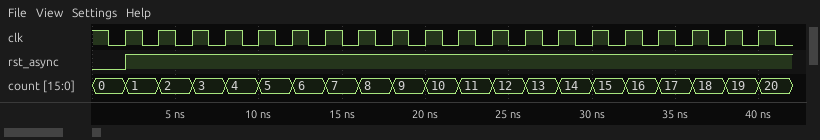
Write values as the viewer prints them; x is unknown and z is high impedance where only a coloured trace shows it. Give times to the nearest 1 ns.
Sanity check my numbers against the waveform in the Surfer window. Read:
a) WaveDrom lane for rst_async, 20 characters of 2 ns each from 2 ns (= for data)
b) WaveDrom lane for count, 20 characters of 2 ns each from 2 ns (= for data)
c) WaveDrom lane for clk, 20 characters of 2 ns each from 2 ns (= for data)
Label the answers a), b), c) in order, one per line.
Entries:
a) {name: 'rst_async', wave: '1...................'}
b) {name: 'count', wave: '====================', data: '1 2 3 4 5 6 7 8 9 10 11 12 13 14 15 16 17 18 19 20'}
c) {name: 'clk', wave: 'p...................'}
